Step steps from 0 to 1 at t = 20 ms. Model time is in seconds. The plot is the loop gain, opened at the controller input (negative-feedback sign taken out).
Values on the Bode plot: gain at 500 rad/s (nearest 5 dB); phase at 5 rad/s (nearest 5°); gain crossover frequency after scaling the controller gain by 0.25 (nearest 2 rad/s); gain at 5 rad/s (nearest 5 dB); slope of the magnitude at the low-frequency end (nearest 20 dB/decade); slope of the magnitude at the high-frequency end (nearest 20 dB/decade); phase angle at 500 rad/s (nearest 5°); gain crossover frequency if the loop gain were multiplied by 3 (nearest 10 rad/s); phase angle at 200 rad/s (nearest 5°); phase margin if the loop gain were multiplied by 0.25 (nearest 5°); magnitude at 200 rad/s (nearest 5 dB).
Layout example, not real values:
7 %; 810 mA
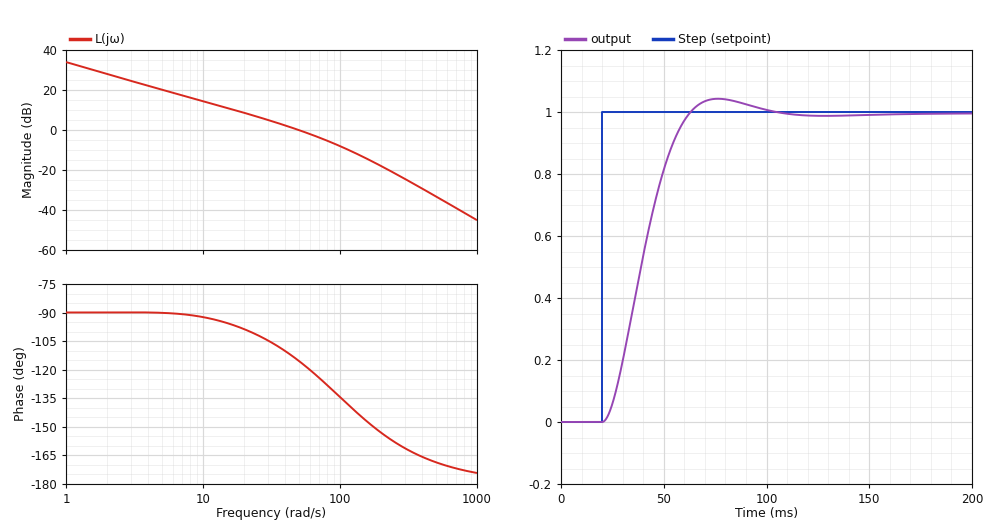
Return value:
-35 dB; -90°; 14 rad/s; 20 dB; -20 dB/decade; -40 dB/decade; -170°; 110 rad/s; -155°; 85°; -20 dB
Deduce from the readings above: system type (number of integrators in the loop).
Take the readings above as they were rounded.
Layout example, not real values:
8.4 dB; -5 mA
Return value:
1
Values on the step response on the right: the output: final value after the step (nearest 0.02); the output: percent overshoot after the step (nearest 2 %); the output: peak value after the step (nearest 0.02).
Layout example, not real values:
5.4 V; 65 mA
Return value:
1.00; 4 %; 1.04
